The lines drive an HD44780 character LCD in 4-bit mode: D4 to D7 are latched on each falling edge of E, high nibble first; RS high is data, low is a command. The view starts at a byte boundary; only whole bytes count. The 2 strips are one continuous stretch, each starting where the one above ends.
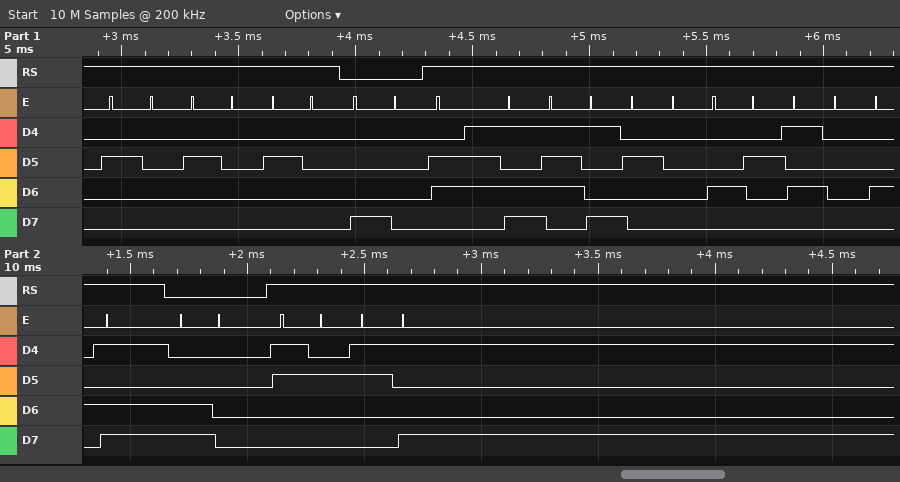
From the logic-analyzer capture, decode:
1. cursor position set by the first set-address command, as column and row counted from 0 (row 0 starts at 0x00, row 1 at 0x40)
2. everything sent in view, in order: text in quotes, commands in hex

column 0, row 0
"   " 0x80 "my BPM" 0xC0 "29"
